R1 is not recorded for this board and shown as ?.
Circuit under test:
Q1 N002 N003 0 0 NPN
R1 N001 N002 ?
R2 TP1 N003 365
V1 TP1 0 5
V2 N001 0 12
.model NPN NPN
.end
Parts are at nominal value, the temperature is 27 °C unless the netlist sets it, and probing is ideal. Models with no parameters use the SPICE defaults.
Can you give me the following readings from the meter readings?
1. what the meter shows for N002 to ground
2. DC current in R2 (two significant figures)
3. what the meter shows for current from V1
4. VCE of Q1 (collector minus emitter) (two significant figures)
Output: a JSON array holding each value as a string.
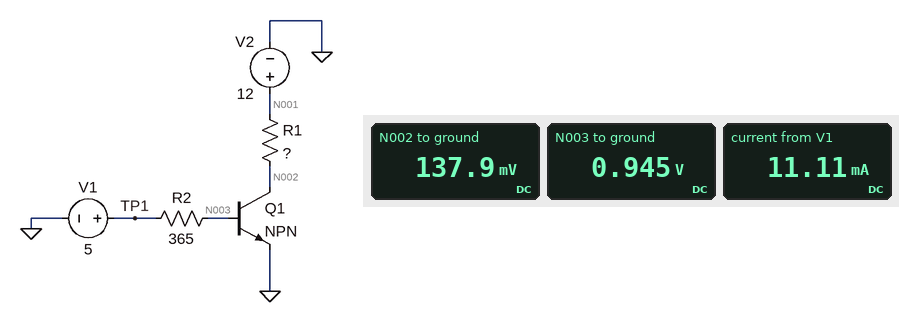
["137.9 mV", "11 mA", "11.11 mA", "140 mV"]
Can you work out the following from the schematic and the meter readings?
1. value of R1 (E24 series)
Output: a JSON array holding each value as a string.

["16 Ω"]
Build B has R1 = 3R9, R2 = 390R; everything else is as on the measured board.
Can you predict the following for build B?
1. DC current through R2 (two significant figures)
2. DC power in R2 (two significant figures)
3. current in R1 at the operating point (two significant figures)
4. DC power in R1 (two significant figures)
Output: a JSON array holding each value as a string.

["10 mA", "42 mW", "1.0 A", "4.2 W"]
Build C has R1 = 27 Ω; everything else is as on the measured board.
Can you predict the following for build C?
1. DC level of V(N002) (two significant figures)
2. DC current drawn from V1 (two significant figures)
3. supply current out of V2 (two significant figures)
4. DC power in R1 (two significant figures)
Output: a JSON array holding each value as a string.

["110 mV", "11 mA", "440 mA", "5.2 W"]
